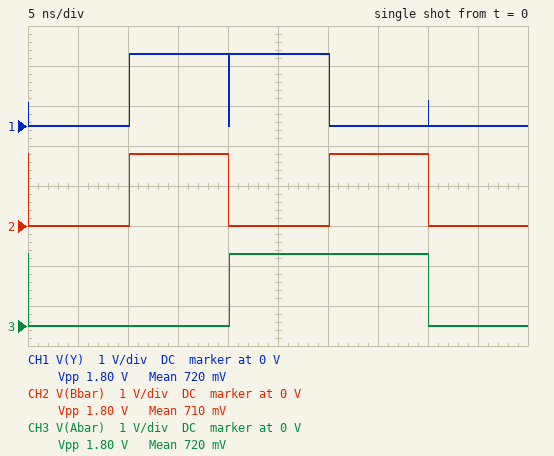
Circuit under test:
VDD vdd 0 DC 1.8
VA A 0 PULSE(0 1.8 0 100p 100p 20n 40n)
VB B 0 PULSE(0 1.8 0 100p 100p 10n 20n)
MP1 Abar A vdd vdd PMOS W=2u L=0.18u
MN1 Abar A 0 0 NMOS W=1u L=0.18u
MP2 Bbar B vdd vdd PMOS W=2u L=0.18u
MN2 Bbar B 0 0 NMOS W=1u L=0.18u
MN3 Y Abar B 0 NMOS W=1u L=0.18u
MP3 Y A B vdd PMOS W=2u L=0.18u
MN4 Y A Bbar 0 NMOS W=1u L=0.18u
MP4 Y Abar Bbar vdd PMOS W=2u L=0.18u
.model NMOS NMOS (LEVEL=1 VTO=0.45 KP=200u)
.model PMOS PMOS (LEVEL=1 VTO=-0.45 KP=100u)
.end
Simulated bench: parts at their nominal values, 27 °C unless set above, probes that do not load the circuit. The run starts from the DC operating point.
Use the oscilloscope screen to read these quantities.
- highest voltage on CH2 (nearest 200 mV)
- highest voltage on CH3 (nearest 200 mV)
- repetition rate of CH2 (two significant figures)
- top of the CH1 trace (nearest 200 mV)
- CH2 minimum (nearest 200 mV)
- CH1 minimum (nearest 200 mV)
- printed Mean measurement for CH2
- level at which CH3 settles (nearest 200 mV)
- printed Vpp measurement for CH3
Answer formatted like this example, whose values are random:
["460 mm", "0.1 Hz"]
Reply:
["1.8 V", "1.8 V", "50 MHz", "1.8 V", "0 V", "0 V", "710 mV", "0 V", "1.80 V"]
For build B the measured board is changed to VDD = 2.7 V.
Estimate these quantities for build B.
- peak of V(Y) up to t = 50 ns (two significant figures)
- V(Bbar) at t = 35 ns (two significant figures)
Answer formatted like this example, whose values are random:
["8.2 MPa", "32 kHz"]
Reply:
["2.6 V", "2.7 V"]
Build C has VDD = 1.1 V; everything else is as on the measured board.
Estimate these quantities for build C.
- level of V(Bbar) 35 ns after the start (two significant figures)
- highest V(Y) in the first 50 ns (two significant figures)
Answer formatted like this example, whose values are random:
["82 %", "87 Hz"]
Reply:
["1.1 V", "1.7 V"]
